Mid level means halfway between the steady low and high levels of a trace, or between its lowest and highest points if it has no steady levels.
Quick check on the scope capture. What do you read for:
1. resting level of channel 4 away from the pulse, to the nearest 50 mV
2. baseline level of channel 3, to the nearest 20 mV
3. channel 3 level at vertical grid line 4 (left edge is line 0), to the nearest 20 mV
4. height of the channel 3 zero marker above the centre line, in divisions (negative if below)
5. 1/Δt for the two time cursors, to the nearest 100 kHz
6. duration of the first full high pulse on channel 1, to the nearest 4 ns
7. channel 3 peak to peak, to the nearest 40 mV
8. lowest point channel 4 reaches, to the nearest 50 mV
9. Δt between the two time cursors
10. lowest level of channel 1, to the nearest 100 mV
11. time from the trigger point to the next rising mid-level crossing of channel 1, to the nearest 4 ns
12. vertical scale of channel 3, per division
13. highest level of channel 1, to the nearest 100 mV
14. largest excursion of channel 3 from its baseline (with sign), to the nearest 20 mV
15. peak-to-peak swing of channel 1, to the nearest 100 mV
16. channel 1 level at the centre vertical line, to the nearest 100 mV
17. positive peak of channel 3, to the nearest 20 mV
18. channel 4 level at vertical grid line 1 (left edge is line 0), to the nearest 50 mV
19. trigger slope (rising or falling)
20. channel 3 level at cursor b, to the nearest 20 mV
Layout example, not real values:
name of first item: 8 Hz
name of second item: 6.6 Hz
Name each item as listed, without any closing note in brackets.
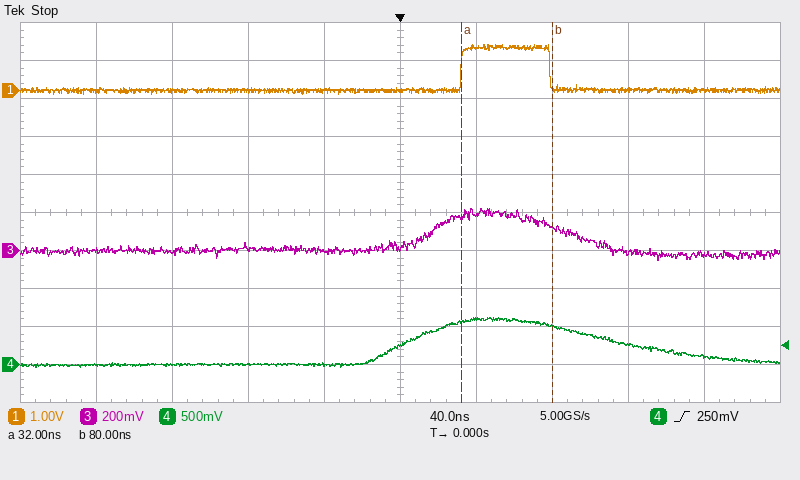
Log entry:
resting level of channel 4 away from the pulse, to the nearest 50 mV: 0 mV
baseline level of channel 3, to the nearest 20 mV: 0 mV
channel 3 level at vertical grid line 4 (left edge is line 0), to the nearest 20 mV: 0 mV
height of the channel 3 zero marker above the centre line, in divisions: -1.0 div
1/Δt for the two time cursors, to the nearest 100 kHz: 20.8 MHz
duration of the first full high pulse on channel 1, to the nearest 4 ns: 48 ns
channel 3 peak to peak, to the nearest 40 mV: 280 mV
lowest point channel 4 reaches, to the nearest 50 mV: -50 mV
Δt between the two time cursors: 48 ns
lowest level of channel 1, to the nearest 100 mV: -100 mV
time from the trigger point to the next rising mid-level crossing of channel 1, to the nearest 4 ns: 32 ns
vertical scale of channel 3, per division: 200 mV
highest level of channel 1, to the nearest 100 mV: 1.2 V
largest excursion of channel 3 from its baseline (with sign), to the nearest 20 mV: +220 mV
peak-to-peak swing of channel 1, to the nearest 100 mV: 1.3 V
channel 1 level at the centre vertical line, to the nearest 100 mV: 0.0 V
positive peak of channel 3, to the nearest 20 mV: 220 mV
channel 4 level at vertical grid line 1 (left edge is line 0), to the nearest 50 mV: 0 mV
trigger slope: rising
channel 3 level at cursor b, to the nearest 20 mV: 120 mV
